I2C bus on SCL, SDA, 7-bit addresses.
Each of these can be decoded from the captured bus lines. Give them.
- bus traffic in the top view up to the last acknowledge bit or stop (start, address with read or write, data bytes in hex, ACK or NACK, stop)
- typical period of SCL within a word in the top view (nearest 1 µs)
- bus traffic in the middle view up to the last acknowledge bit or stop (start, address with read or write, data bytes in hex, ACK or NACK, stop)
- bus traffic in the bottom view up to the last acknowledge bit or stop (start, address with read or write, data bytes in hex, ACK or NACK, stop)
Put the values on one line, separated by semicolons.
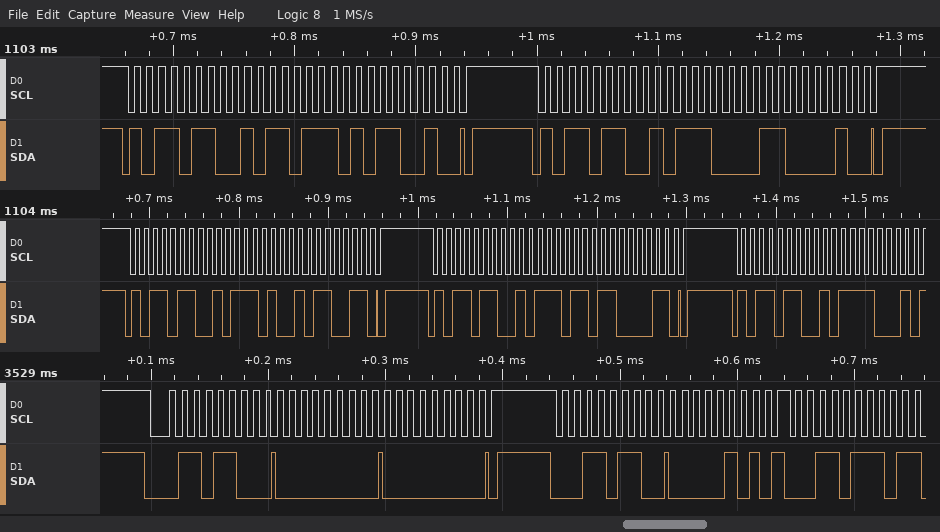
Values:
start, address 5B write ACK, B7 ACK, B2 ACK, stop, start, address 5B write ACK, B8 ACK, C2 ACK, stop; 10 µs; start, address 5B write ACK, BA ACK, B3 ACK, stop, start, address 5B write ACK, BB ACK, C3 ACK, stop, start, address 5B write ACK, BC ACK; start, address 36 write ACK, 00 ACK, 00 ACK, stop, start, address 1B write ACK, 05 ACK, repeated start, address 1B read ACK
